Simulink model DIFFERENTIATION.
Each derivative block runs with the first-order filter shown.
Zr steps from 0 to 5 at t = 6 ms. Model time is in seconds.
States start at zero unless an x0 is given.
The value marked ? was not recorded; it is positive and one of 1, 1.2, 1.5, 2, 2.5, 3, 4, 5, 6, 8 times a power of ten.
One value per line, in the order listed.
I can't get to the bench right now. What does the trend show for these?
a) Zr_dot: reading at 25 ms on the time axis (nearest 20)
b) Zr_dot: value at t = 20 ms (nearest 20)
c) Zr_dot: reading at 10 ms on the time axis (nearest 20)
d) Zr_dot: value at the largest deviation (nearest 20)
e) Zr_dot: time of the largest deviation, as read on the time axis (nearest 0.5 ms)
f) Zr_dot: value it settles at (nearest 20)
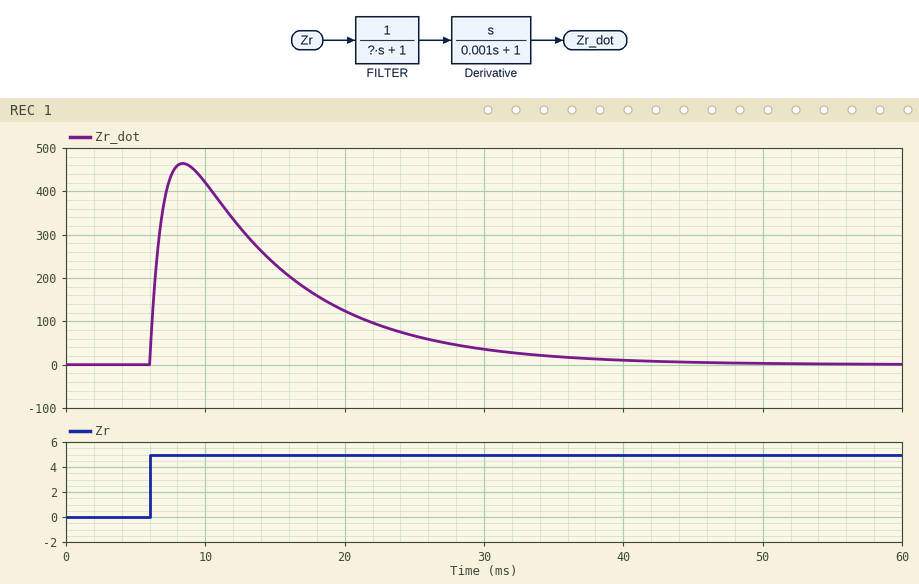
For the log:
60
120
420
460
8.5 ms
0
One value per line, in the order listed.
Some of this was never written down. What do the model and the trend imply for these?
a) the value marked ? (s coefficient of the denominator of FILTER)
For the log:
0.008
